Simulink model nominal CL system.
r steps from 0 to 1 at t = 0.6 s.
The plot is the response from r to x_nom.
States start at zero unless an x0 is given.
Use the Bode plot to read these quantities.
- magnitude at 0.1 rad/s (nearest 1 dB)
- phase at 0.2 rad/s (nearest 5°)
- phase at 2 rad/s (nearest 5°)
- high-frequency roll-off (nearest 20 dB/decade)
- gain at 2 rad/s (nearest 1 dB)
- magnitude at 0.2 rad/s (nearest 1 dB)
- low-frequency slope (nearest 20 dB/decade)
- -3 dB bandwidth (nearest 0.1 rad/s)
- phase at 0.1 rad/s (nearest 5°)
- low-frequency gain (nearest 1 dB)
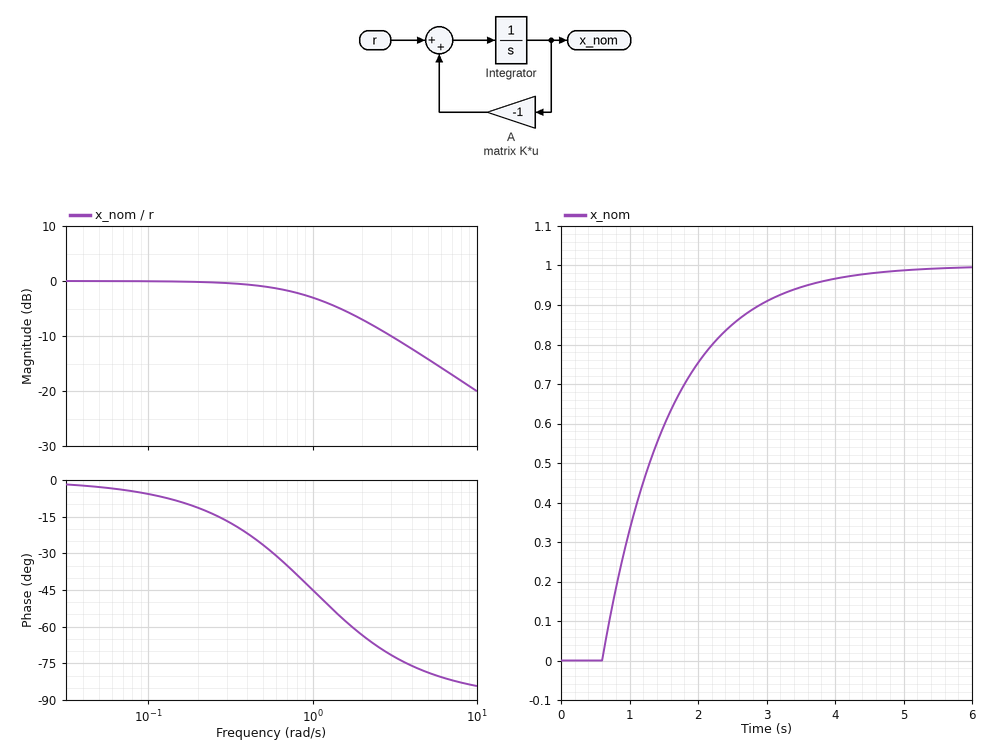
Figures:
0 dB
-10°
-65°
-20 dB/decade
-7 dB
0 dB
0 dB/decade
1.0 rad/s
-5°
0 dB
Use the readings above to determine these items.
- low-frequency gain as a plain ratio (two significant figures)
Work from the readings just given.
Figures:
1.0
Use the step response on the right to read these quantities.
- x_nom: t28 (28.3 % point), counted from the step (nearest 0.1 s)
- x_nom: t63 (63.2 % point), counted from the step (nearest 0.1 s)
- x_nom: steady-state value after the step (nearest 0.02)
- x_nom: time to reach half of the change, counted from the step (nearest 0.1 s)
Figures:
0.3 s
1.0 s
1.00
0.7 s
